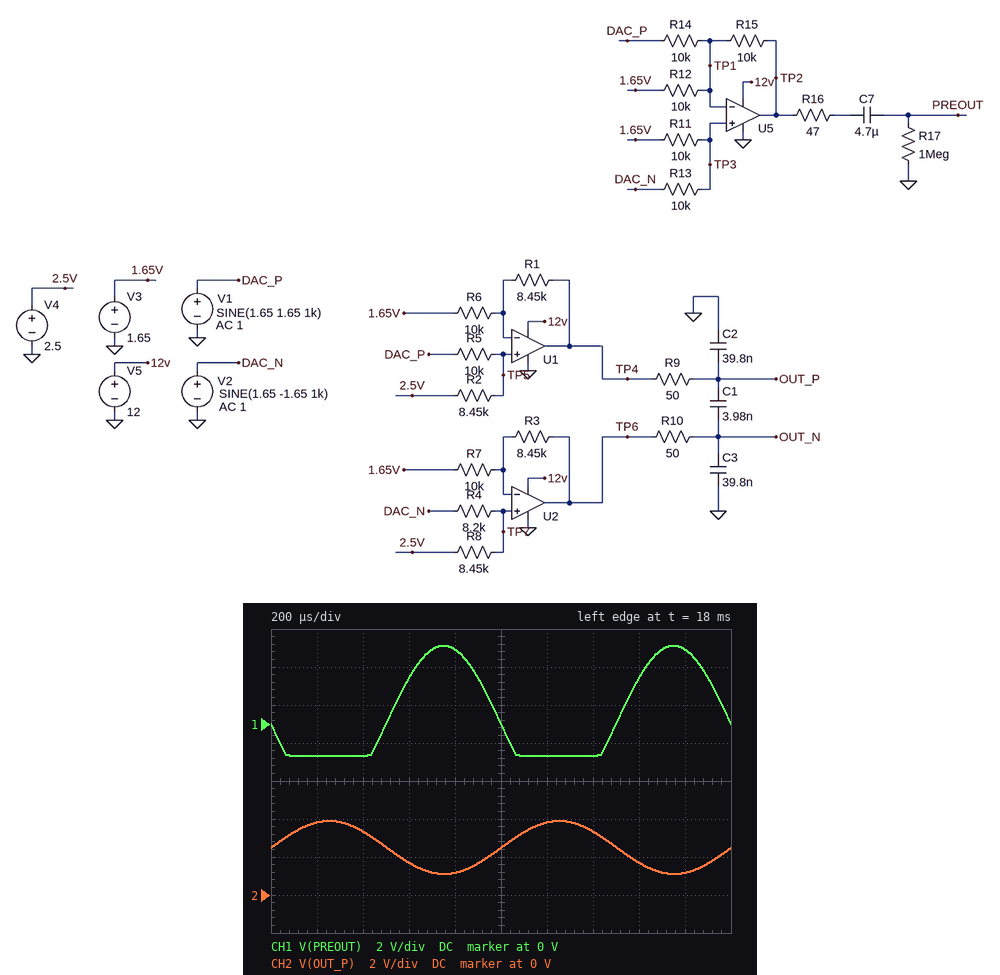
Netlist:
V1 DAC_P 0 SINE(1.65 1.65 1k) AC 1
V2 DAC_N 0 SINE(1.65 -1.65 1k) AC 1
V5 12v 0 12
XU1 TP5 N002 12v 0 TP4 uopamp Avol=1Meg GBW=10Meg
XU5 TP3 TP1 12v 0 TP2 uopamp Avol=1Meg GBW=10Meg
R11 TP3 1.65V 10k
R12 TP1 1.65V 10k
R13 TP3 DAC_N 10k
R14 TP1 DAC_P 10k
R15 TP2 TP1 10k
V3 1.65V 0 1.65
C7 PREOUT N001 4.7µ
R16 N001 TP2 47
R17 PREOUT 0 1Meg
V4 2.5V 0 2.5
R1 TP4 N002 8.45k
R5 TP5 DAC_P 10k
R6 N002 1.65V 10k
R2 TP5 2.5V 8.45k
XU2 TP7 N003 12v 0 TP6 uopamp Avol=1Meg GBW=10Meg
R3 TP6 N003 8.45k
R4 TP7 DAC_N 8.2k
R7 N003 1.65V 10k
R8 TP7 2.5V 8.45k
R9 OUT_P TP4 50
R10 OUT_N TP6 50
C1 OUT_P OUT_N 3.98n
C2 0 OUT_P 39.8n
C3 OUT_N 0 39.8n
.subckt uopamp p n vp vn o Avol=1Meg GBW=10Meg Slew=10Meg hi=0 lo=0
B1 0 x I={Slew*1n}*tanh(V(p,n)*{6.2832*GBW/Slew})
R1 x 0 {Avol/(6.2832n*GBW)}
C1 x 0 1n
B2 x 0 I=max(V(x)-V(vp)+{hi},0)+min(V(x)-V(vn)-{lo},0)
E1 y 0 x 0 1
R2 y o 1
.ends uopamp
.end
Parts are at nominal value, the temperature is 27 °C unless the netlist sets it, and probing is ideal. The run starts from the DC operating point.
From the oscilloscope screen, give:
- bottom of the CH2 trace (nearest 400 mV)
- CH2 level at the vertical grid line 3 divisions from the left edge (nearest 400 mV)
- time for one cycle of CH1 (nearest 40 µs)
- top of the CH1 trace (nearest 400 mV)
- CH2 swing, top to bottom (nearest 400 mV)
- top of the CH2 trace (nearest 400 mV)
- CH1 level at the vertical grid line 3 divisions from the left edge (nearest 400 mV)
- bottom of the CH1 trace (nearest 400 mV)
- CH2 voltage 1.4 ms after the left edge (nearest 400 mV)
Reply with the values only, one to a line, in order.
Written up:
1.2 V
1.6 V
1.00 ms
4.0 V
2.8 V
4.0 V
2.4 V
-1.6 V
3.2 V
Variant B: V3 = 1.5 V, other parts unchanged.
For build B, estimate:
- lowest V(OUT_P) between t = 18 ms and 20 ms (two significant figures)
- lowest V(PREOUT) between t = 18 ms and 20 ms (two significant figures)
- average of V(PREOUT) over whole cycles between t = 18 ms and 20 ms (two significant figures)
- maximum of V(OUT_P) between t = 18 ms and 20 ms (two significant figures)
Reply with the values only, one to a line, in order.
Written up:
1.2 V
-1.6 V
620 mV
4.0 V
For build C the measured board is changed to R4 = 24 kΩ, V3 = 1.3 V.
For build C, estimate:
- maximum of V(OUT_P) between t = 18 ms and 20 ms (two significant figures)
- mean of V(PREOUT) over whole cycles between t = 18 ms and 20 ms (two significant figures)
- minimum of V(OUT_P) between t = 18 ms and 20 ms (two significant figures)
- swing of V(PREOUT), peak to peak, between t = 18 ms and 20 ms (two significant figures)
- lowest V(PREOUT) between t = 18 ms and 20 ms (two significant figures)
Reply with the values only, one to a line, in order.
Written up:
4.2 V
650 mV
1.4 V
5.6 V
-1.5 V
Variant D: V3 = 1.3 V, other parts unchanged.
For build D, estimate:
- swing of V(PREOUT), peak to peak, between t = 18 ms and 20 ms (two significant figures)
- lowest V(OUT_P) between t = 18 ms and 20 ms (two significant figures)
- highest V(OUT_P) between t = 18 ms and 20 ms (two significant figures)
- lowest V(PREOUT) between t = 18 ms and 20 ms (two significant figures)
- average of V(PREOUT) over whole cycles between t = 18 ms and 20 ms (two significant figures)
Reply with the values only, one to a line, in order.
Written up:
5.6 V
1.4 V
4.2 V
-1.5 V
650 mV
